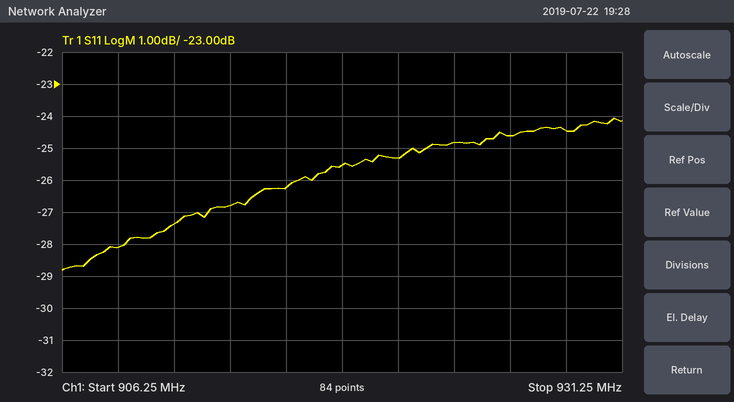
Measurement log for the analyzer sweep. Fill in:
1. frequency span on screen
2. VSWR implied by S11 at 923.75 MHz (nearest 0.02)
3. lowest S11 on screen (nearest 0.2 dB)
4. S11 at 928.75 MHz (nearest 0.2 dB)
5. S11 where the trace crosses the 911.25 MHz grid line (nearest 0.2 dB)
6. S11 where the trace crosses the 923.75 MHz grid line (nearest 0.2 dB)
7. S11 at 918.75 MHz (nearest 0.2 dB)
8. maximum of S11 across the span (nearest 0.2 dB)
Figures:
25 MHz
1.12
-28.8 dB
-24.4 dB
-27.4 dB
-24.8 dB
-25.6 dB
-24.0 dB
